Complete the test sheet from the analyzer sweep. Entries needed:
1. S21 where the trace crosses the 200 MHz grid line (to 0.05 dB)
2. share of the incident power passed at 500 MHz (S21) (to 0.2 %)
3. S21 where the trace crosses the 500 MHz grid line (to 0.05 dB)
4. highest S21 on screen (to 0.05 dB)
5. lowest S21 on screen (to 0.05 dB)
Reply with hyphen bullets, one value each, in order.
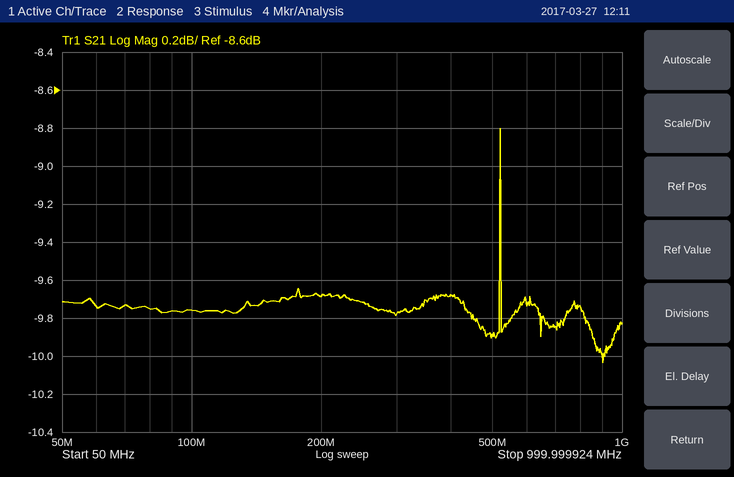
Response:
- -9.70 dB
- 10.2 %
- -9.90 dB
- -8.80 dB
- -10.05 dB
